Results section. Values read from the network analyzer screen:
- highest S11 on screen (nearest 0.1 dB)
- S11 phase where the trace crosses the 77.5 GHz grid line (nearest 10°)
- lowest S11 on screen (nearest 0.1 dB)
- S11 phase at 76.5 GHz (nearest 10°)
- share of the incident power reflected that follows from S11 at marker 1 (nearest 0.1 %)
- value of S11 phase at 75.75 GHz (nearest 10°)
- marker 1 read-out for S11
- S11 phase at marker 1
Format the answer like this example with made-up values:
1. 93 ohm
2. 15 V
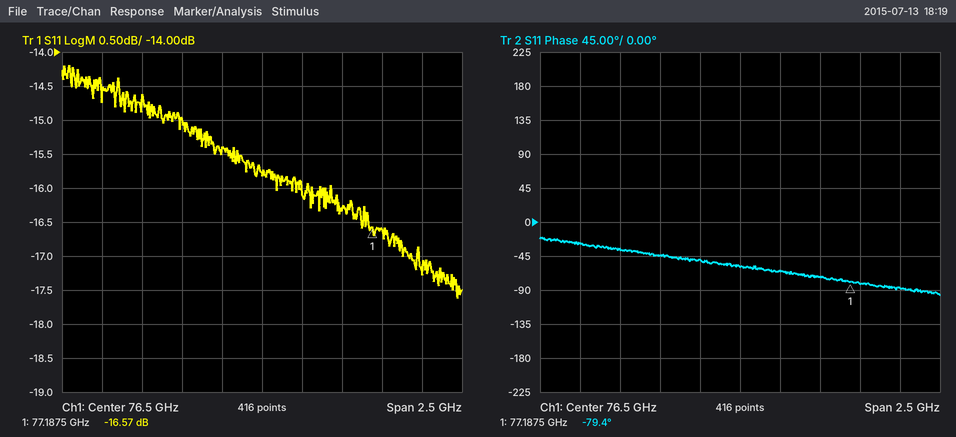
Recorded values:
1. -14.2 dB
2. -90°
3. -17.6 dB
4. -60°
5. 2.2 %
6. -40°
7. -16.57 dB
8. -79.4°
